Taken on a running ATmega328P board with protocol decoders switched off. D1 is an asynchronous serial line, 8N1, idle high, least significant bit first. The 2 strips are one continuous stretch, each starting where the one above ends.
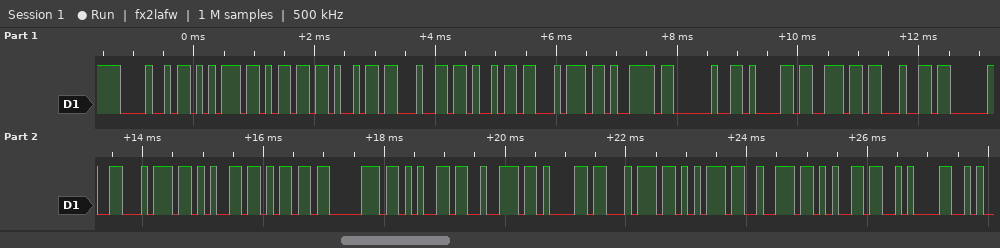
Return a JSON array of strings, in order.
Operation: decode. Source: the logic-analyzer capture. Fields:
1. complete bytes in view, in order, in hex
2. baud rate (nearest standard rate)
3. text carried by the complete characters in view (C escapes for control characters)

["48 75 6D 69 64 69 74 79 20 61 6E 64 20 74 65 6D 70 65 72 61 74 75 72 65 0A", "9600 baud", "\"Humidity and temperature\\n\""]
